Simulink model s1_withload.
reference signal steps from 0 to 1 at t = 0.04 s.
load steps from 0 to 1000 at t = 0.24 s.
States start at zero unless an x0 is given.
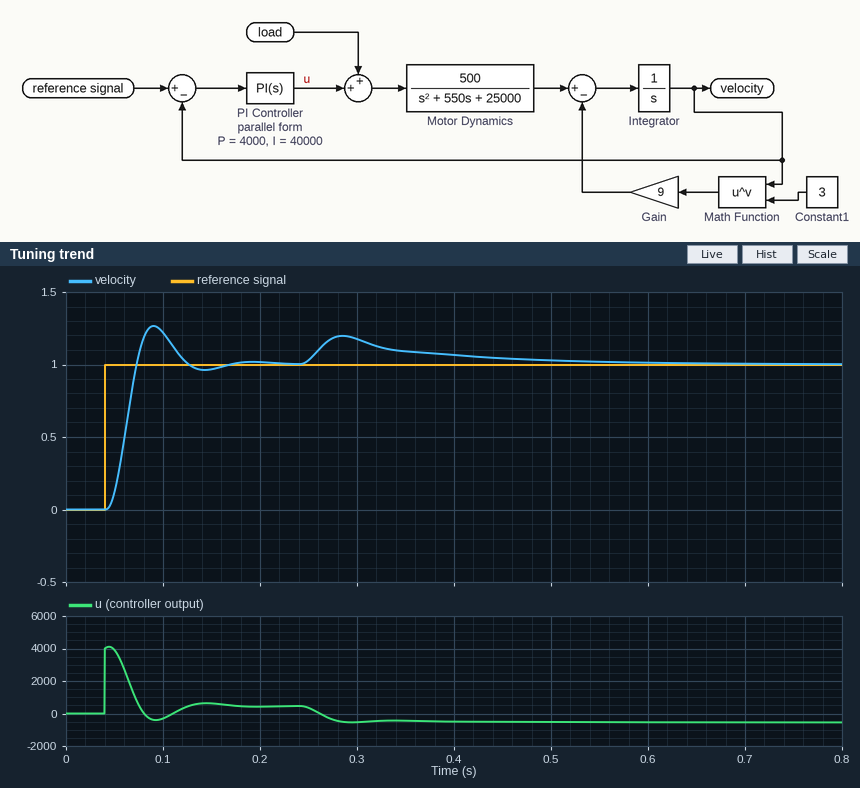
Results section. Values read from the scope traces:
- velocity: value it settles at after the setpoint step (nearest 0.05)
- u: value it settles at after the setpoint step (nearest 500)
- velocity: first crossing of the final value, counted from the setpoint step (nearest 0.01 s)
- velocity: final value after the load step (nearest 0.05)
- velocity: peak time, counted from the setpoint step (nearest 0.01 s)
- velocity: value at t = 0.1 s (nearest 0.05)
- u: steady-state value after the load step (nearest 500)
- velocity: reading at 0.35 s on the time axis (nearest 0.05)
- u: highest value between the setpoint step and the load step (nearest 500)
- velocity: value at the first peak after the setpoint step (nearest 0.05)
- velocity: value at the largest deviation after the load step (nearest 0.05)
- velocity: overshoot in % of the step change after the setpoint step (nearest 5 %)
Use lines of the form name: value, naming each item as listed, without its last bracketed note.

velocity: value it settles at after the setpoint step: 1.00
u: value it settles at after the setpoint step: 500
velocity: first crossing of the final value, counted from the setpoint step: 0.03 s
velocity: final value after the load step: 1.00
velocity: peak time, counted from the setpoint step: 0.05 s
velocity: value at t = 0.1 s: 1.20
u: steady-state value after the load step: -500
velocity: reading at 0.35 s on the time axis: 1.10
u: highest value between the setpoint step and the load step: 4000
velocity: value at the first peak after the setpoint step: 1.25
velocity: value at the largest deviation after the load step: 1.20
velocity: overshoot in % of the step change after the setpoint step: 25 %
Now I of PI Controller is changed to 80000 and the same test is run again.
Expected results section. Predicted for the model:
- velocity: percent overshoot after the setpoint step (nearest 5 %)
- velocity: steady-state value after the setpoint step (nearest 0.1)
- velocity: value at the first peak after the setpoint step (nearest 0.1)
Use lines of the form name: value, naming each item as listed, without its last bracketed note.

velocity: percent overshoot after the setpoint step: 40 %
velocity: steady-state value after the setpoint step: 1.0
velocity: value at the first peak after the setpoint step: 1.4
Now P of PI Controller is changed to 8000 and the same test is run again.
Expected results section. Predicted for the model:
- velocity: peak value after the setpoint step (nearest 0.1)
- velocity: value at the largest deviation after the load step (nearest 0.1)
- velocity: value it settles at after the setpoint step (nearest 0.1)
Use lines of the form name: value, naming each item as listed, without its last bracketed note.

velocity: peak value after the setpoint step: 1.4
velocity: value at the largest deviation after the load step: 1.1
velocity: value it settles at after the setpoint step: 1.0
